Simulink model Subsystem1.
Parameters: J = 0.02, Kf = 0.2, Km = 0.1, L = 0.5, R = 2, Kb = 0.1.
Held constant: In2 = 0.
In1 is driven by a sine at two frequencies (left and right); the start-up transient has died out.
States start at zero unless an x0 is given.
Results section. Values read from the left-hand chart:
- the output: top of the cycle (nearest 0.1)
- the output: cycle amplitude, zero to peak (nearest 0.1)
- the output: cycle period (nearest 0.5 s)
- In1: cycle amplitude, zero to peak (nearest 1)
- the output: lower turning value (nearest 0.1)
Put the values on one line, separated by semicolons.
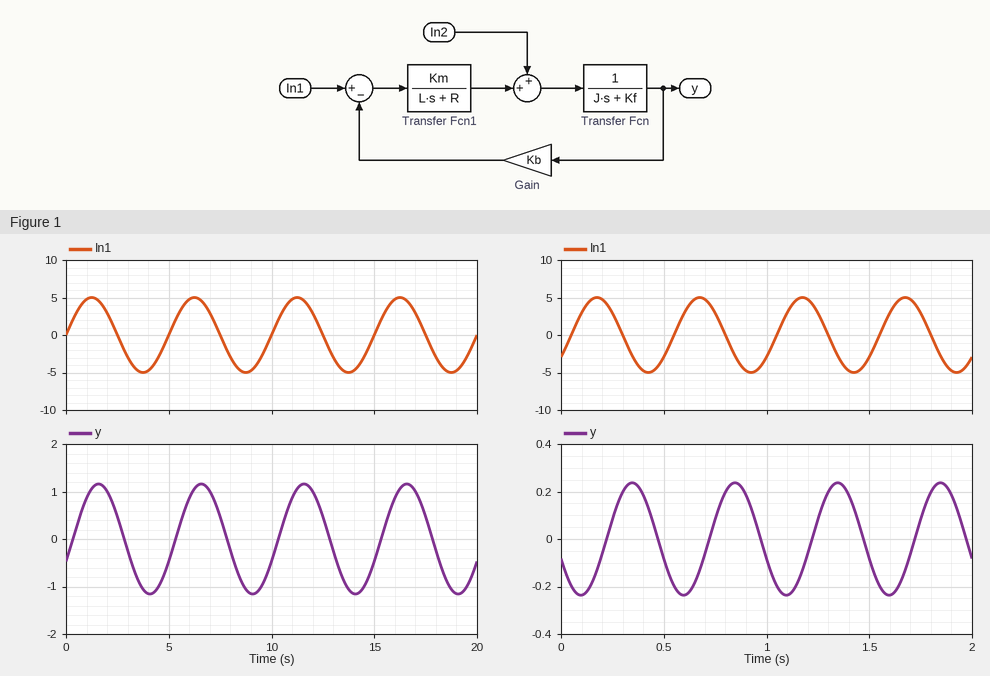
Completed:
1.2; 1.2; 5.0 s; 5; -1.2
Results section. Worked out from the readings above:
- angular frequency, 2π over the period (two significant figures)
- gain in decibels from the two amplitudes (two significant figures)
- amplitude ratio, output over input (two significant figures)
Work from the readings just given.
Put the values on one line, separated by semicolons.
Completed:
1.3 rad/s; -12 dB; 0.24
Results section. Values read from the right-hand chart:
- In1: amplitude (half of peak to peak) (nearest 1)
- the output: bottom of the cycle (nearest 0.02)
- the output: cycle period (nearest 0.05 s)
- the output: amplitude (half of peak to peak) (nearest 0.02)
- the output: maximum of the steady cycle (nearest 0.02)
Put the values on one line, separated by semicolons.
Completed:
5; -0.24; 0.50 s; 0.24; 0.24
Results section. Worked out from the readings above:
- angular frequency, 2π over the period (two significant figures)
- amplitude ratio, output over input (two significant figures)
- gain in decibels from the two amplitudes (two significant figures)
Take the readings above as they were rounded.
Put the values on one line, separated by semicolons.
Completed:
13 rad/s; 0.048; -26 dB
